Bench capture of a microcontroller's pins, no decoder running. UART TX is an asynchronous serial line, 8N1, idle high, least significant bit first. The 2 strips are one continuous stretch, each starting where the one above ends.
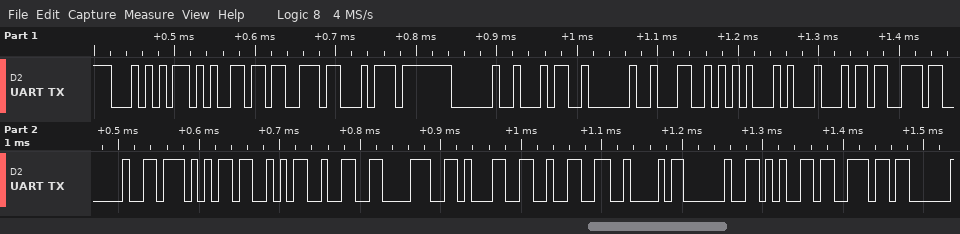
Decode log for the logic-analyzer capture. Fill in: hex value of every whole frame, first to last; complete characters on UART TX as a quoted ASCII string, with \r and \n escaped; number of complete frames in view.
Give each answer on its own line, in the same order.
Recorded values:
54 65 73 74 20 34 20 4C 45 44 73 20 57 53 32 38 31 32 42 20 65 6E
"Test 4 LEDs WS2812B en"
22
